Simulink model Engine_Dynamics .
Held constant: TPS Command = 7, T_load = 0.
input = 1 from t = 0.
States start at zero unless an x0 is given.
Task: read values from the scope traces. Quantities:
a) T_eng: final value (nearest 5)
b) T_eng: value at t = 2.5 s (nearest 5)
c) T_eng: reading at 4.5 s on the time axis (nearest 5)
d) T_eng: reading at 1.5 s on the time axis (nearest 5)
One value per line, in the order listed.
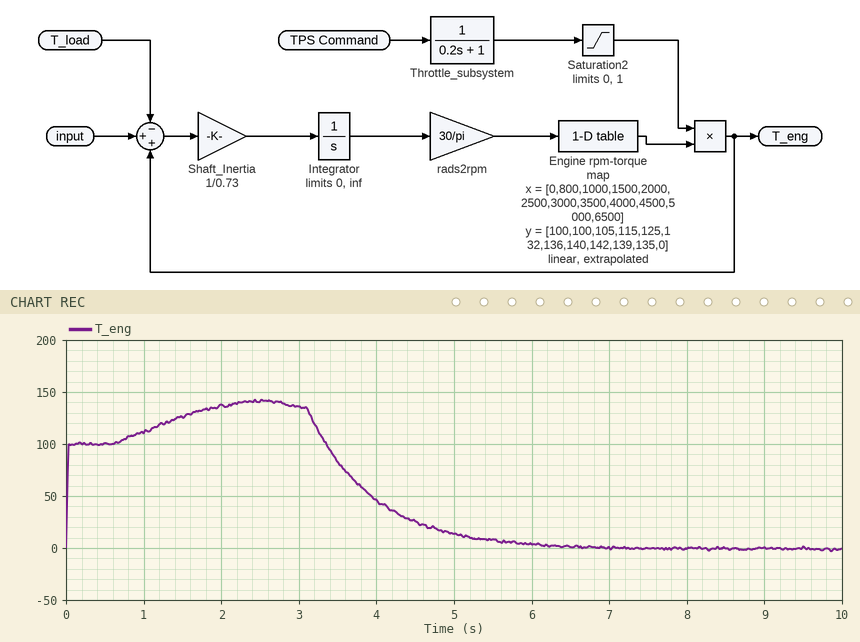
0
140
25
125
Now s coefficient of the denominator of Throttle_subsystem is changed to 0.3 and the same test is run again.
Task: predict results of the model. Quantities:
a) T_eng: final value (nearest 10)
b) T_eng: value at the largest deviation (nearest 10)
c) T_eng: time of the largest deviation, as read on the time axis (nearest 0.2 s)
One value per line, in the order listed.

0
140
2.6 s
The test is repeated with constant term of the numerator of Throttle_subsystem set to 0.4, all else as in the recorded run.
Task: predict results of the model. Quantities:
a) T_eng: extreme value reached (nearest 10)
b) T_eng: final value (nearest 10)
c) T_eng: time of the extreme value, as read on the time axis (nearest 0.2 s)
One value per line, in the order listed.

140
0
2.6 s
